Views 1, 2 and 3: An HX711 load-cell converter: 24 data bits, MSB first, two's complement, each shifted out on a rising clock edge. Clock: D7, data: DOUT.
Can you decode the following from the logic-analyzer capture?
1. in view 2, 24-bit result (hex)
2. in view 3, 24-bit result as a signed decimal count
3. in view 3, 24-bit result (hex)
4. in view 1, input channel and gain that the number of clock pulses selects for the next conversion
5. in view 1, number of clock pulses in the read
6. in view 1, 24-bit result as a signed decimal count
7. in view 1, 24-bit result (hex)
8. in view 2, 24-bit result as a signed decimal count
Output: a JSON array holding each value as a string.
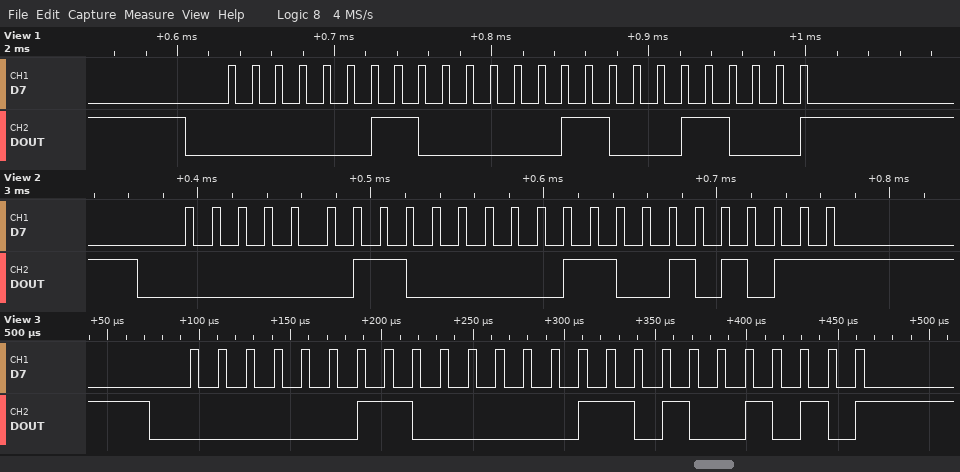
["0x03032B", "197450", "0x03034A", "channel A, gain 128", "25", "197400", "0x030318", "197419"]
